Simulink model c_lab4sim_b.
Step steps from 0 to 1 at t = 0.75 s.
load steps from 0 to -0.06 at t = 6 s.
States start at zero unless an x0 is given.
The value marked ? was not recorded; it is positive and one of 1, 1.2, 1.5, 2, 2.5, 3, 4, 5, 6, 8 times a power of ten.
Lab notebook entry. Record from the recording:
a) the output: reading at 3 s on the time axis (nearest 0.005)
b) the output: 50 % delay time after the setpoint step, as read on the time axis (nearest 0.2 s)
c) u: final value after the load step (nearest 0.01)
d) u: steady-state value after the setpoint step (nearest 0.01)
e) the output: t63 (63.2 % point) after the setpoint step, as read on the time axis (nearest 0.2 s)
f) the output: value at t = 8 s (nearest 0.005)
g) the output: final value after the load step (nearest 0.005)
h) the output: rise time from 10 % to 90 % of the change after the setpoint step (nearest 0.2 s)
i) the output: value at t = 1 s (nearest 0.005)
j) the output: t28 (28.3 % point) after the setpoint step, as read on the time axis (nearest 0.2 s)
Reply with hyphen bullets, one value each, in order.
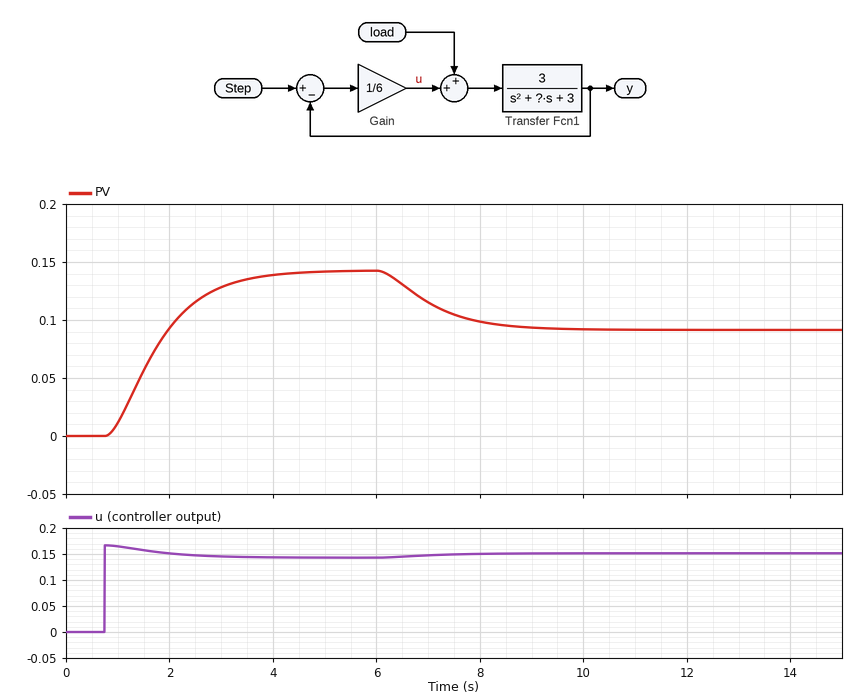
- 0.130
- 1.6 s
- 0.15
- 0.14
- 2.0 s
- 0.100
- 0.090
- 2.0 s
- 0.010
- 1.4 s
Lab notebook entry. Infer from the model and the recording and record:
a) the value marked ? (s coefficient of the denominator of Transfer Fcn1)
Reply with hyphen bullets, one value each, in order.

- 4
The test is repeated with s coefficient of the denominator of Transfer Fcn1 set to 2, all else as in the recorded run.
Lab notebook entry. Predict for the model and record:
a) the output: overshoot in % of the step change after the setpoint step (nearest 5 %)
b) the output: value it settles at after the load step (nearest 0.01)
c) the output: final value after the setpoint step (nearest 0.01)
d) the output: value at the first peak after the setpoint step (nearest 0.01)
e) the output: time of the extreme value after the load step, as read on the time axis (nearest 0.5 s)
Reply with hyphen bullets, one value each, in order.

- 15 %
- 0.09
- 0.14
- 0.16
- 8.0 s
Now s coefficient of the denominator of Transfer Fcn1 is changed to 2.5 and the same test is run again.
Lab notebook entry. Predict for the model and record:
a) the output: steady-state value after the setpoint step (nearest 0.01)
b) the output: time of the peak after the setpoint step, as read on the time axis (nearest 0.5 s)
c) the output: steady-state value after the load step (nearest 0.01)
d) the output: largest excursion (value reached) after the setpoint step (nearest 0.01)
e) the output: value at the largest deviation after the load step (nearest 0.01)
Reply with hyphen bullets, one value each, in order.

- 0.14
- 3.0 s
- 0.09
- 0.15
- 0.09
